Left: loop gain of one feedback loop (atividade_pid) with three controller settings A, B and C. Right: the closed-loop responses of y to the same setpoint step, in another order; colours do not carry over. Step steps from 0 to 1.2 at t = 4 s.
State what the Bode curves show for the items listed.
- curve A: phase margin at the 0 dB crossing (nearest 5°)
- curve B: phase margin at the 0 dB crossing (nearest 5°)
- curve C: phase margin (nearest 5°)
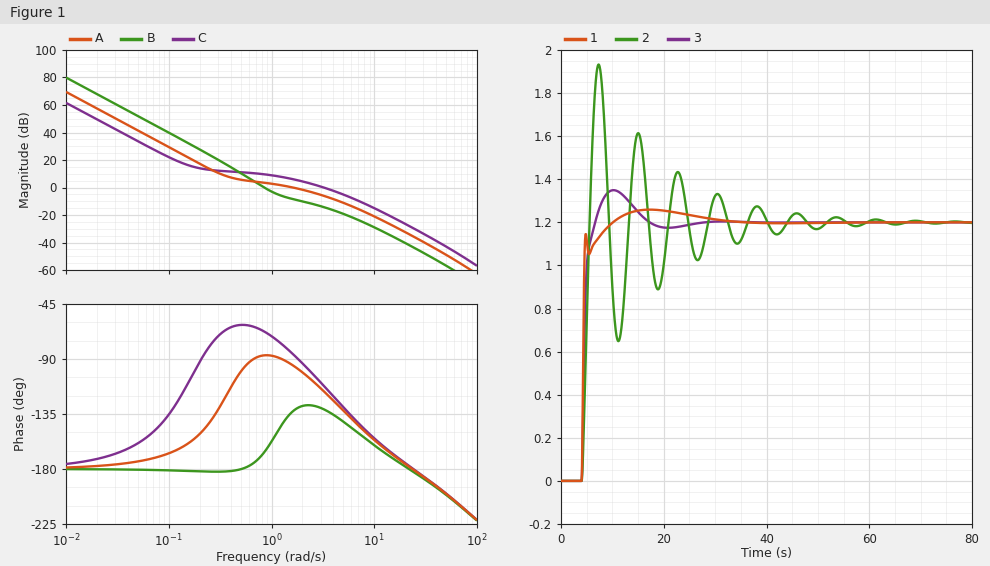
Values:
85°
15°
70°
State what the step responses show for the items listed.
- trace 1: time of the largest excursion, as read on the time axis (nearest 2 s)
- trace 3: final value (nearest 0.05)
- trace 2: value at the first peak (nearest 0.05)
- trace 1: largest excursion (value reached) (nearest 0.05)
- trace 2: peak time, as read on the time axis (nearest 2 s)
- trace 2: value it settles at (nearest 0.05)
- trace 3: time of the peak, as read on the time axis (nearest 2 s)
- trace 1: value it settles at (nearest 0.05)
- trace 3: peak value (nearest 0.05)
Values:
18 s
1.20
1.95
1.25
8 s
1.20
10 s
1.20
1.35
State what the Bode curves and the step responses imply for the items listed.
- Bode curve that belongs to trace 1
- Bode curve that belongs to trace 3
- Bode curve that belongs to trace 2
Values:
C
A
B
